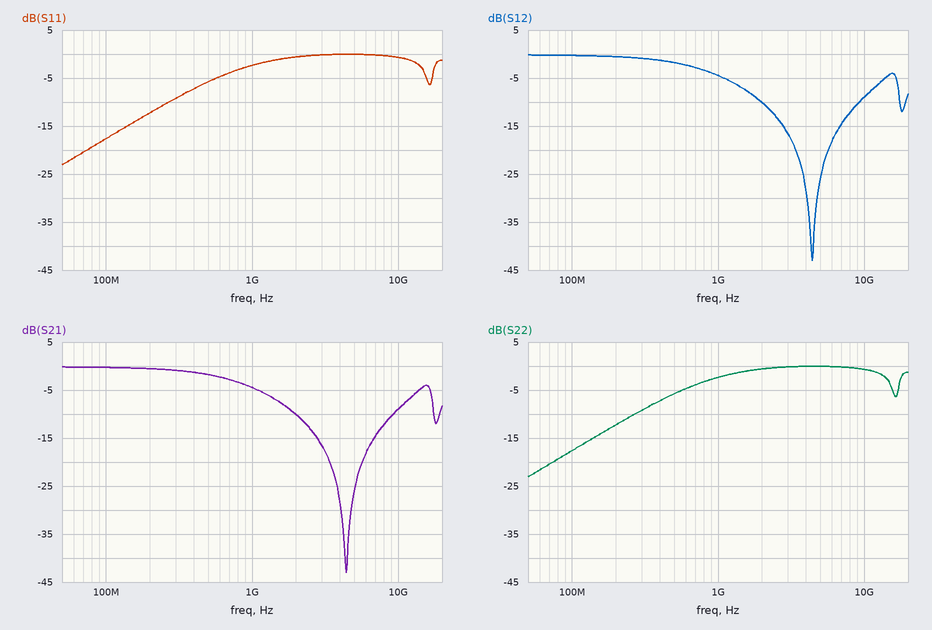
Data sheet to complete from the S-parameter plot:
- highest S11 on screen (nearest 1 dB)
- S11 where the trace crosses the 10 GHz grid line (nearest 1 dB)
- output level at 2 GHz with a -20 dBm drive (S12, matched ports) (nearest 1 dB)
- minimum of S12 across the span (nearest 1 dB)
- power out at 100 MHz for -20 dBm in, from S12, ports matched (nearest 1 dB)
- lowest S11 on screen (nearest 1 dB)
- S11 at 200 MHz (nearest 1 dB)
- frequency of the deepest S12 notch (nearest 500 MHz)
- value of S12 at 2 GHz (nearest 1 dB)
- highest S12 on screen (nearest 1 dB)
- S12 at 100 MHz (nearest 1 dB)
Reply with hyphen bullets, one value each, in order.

- 0 dB
- -1 dB
- -30 dBm
- -43 dB
- -20 dBm
- -23 dB
- -12 dB
- 4.5 GHz
- -10 dB
- 0 dB
- 0 dB
